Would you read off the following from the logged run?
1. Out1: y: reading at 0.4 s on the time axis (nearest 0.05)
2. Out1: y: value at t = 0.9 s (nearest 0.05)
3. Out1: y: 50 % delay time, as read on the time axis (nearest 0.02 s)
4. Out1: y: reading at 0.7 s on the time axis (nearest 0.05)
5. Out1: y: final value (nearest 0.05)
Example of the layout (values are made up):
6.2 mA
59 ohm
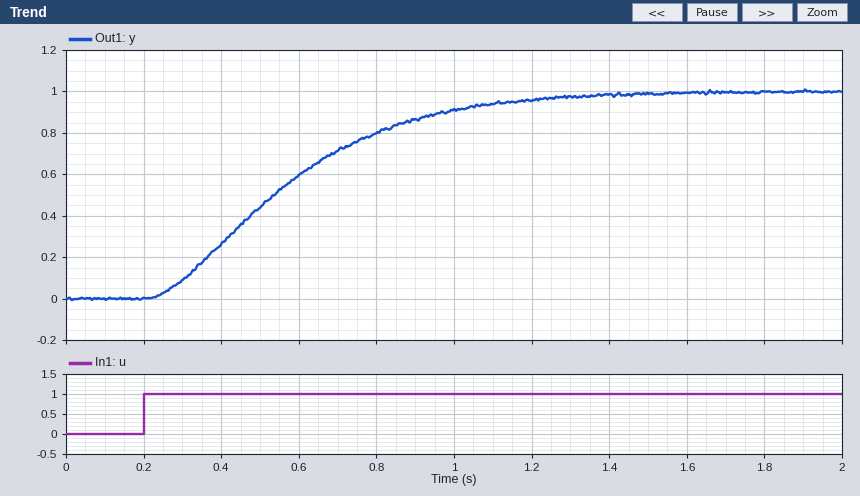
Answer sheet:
0.25
0.85
0.54 s
0.70
1.00
